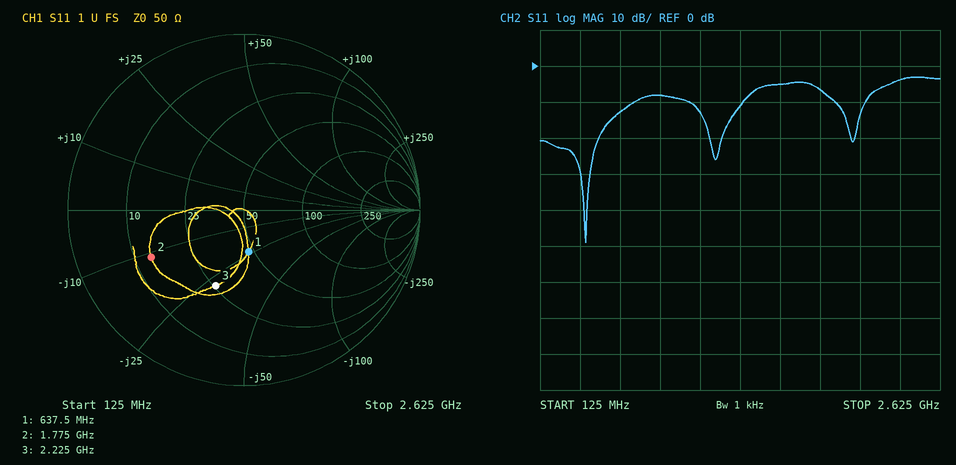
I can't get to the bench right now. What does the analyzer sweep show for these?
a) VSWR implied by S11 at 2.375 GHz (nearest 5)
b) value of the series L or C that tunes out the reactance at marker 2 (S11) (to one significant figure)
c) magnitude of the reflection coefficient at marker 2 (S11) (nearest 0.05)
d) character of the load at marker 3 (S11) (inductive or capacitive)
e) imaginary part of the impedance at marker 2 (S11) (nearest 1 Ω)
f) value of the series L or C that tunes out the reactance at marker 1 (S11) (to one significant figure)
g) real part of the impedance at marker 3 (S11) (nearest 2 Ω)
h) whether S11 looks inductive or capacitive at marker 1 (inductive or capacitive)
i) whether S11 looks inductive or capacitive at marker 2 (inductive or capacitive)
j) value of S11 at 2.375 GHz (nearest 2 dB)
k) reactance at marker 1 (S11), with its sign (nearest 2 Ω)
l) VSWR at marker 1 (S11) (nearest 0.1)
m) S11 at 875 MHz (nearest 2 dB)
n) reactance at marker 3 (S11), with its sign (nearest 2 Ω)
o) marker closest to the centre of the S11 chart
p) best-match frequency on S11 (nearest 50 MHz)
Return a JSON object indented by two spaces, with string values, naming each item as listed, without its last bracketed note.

{
  "VSWR implied by S11 at 2.375 GHz": "5",
  "value of the series L or C that tunes out the reactance at marker 2 (S11)": "1.0 nH",
  "magnitude of the reflection coefficient at marker 2 (S11)": "0.60",
  "character of the load at marker 3 (S11)": "capacitive",
  "imaginary part of the impedance at marker 2 (S11)": "-11 Ω",
  "value of the series L or C that tunes out the reactance at marker 1 (S11)": "6 nH",
  "real part of the impedance at marker 3 (S11)": "26 Ω",
  "whether S11 looks inductive or capacitive at marker 1": "capacitive",
  "whether S11 looks inductive or capacitive at marker 2": "capacitive",
  "value of S11 at 2.375 GHz": "-4 dB",
  "reactance at marker 1 (S11), with its sign": "-24 Ω",
  "VSWR at marker 1 (S11)": "1.6",
  "S11 at 875 MHz": "-8 dB",
  "reactance at marker 3 (S11), with its sign": "-28 Ω",
  "marker closest to the centre of the S11 chart": "marker 1",
  "best-match frequency on S11": "400 MHz"
}
